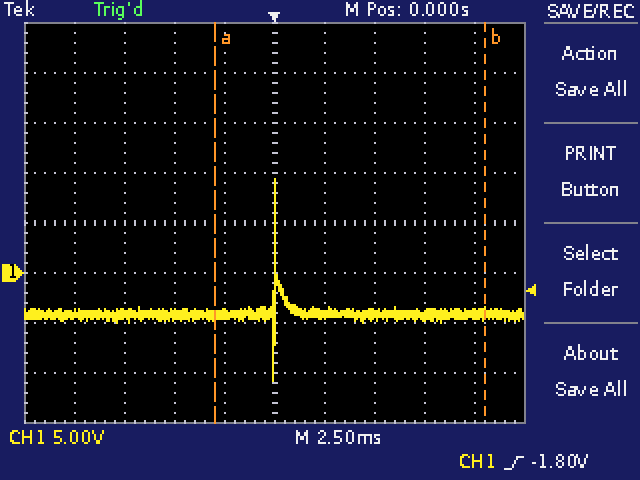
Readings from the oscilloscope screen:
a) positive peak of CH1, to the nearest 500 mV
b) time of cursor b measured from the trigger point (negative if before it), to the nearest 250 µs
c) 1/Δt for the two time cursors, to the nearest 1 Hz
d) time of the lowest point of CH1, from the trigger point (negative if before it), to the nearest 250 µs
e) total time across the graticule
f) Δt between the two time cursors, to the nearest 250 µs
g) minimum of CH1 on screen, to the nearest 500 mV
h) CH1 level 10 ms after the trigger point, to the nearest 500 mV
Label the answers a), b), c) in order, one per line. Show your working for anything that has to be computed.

a) 9.5 V
b) +10.50 ms
c) 1 / 13.50 ms ≈ 74 Hz
d) 0.00 ms
e) 25 ms
f) 13.50 ms
g) -11.0 V
h) -4.0 V
